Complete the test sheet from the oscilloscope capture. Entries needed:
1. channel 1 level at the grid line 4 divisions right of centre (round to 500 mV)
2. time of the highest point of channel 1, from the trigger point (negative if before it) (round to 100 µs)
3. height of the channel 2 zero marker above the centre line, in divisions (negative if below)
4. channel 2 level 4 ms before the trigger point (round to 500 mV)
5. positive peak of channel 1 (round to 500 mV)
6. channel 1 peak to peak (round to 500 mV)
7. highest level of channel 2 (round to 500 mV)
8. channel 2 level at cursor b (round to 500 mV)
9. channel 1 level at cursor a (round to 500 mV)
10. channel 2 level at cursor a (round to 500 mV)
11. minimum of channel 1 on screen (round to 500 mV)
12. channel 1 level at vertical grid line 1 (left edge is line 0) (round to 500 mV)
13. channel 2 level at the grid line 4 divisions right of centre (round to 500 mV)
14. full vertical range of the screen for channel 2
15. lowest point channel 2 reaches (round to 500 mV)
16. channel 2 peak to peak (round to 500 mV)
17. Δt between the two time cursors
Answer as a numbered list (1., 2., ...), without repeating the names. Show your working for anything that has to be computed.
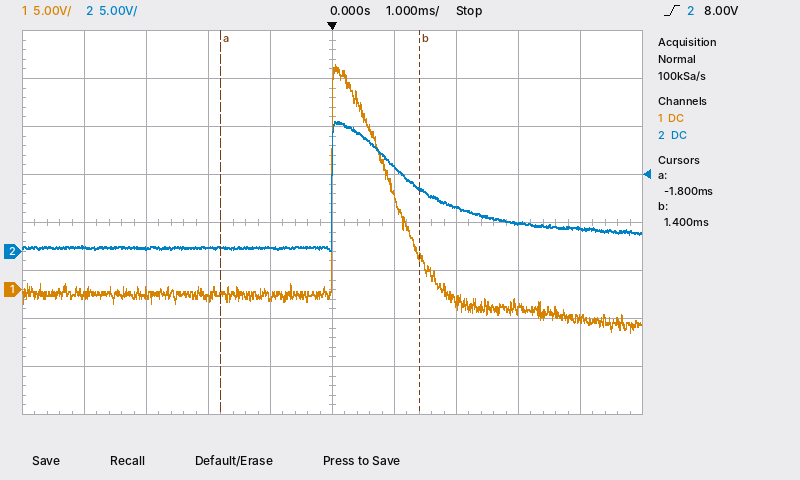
1. -3.0 V
2. +100 µs
3. -0.6 div
4. 500 mV
5. 23.5 V
6. 23.5 V − (-4.5 V) = 28.0 V
7. 13.5 V
8. 6.5 V
9. -500 mV
10. 500 mV
11. -4.5 V
12. -500 mV
13. 2.5 V
14. 40 V
15. 0.0 V
16. 13.5 V − (0.0 V) = 13.5 V
17. 1.4 ms − (-1.8 ms) = 3.2 ms
